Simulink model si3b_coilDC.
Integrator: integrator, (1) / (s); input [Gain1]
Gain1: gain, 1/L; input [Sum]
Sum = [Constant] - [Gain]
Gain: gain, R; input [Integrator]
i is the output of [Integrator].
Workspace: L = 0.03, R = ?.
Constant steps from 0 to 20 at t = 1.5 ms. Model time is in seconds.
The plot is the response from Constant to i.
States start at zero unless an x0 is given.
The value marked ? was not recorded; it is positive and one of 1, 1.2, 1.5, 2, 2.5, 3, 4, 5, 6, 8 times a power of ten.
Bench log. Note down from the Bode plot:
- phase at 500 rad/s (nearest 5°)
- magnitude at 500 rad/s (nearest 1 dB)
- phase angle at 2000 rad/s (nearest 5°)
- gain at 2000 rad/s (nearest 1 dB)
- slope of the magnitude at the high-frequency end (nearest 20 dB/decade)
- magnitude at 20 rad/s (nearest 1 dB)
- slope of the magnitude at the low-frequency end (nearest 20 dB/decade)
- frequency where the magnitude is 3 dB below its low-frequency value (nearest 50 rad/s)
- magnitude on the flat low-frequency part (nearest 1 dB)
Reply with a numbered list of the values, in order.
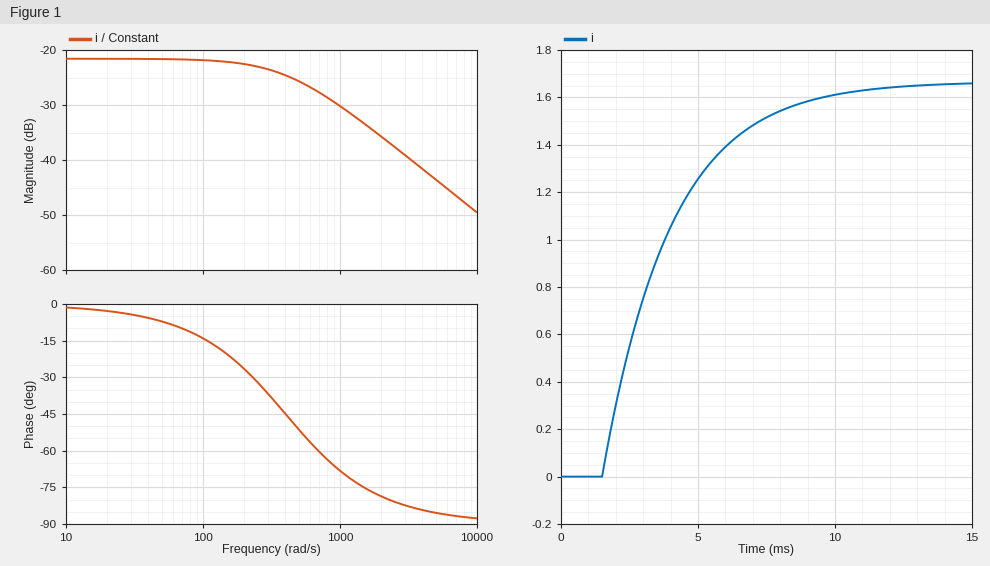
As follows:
1. -50°
2. -26 dB
3. -80°
4. -36 dB
5. -20 dB/decade
6. -22 dB
7. 0 dB/decade
8. 400 rad/s
9. -22 dB
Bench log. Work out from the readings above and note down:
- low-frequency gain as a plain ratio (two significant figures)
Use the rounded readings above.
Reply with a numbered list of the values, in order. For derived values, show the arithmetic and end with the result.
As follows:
1. 10^(-22 / 20) = 0.079
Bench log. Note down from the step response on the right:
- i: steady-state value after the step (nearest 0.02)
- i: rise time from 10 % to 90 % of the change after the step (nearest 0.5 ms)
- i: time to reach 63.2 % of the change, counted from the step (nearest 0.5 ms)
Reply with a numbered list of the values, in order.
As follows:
1. 1.66
2. 5.5 ms
3. 2.5 ms
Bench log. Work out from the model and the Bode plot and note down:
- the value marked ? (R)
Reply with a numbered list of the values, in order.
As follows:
1. 12
